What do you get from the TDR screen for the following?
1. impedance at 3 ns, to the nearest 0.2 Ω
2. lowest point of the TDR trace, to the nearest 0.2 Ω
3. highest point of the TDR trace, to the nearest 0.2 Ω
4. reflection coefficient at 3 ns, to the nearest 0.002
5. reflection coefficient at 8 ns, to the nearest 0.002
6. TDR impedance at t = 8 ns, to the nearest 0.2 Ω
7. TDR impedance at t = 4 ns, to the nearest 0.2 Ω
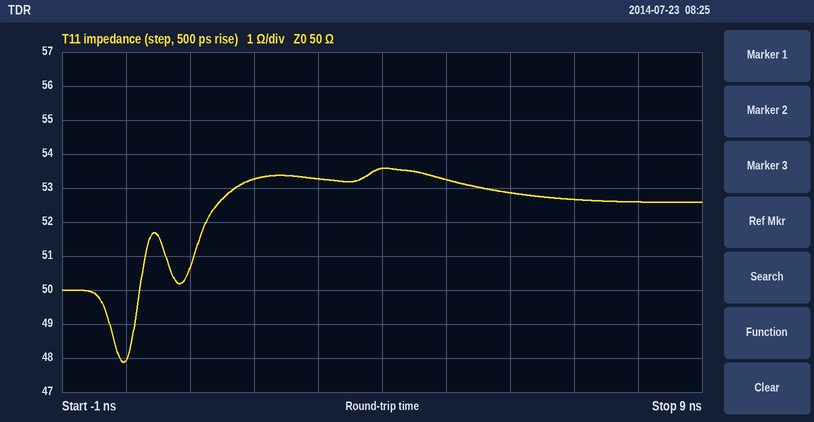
53.2 Ω
47.8 Ω
53.6 Ω
+0.032
+0.026
52.6 Ω
53.6 Ω
